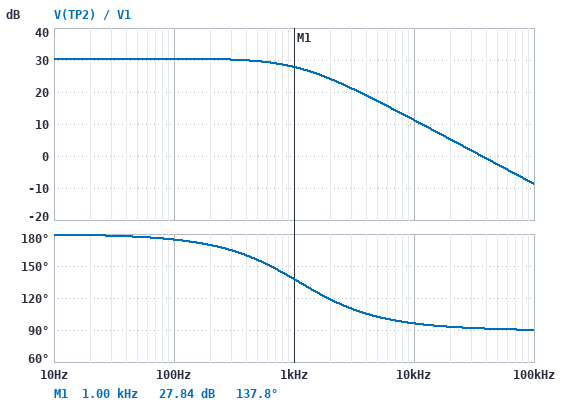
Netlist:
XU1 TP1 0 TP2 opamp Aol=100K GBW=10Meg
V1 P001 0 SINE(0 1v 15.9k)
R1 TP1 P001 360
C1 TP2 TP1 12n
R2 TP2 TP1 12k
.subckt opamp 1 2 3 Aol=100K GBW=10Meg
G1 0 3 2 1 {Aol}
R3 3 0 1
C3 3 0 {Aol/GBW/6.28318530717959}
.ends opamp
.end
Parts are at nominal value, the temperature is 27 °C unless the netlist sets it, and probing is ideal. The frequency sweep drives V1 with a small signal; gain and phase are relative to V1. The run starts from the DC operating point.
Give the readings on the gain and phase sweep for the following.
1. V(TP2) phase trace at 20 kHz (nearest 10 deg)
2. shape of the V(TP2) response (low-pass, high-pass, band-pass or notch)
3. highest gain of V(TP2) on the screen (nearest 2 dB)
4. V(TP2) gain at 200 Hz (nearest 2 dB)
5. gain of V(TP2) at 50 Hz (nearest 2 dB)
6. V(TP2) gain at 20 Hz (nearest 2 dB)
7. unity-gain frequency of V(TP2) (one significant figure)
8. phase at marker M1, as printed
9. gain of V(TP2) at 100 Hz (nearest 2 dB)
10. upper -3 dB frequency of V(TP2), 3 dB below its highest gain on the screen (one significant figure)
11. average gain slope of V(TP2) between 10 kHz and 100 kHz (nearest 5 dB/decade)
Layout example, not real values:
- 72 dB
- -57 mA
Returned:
- 90 deg
- low-pass
- 30 dB
- 30 dB
- 30 dB
- 30 dB
- 40 kHz
- 137.8 deg
- 30 dB
- 1 kHz
- -20 dB/decade
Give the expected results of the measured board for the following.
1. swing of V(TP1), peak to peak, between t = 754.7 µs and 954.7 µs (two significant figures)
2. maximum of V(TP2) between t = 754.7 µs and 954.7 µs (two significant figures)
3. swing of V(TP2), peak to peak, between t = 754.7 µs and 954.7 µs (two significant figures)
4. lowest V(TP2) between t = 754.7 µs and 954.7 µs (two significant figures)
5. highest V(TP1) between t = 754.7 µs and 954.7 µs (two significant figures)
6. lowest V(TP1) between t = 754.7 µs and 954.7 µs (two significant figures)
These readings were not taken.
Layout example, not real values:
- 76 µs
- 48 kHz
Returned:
- 7.3 mV
- 2.3 V
- 4.6 V
- -2.3 V
- 3.7 mV
- -3.7 mV
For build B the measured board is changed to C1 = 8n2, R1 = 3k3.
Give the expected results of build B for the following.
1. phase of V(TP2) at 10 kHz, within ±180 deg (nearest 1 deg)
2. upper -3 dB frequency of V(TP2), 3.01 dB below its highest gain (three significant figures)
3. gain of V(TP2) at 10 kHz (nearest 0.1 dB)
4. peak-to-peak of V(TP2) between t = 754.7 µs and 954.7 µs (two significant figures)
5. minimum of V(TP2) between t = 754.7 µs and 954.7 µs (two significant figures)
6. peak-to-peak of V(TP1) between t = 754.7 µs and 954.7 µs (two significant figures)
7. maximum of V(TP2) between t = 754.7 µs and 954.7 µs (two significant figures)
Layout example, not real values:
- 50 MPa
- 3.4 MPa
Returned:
- 99 deg
- 1.62 kHz
- -4.7 dB
- 740 mV
- -370 mV
- 1.2 mV
- 370 mV
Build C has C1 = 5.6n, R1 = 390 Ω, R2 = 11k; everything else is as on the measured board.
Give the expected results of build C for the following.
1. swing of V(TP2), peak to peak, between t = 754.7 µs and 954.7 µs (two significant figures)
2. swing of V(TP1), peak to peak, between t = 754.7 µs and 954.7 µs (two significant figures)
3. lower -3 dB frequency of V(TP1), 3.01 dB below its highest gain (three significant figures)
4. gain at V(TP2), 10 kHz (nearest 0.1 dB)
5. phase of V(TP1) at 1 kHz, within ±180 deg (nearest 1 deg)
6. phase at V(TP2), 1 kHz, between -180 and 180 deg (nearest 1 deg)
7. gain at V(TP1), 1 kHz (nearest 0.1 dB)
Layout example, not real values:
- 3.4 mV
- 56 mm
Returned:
- 9.0 V
- 14 mV
- 2.56 kHz
- 16.9 dB
- 63 deg
- 159 deg
- -51.6 dB
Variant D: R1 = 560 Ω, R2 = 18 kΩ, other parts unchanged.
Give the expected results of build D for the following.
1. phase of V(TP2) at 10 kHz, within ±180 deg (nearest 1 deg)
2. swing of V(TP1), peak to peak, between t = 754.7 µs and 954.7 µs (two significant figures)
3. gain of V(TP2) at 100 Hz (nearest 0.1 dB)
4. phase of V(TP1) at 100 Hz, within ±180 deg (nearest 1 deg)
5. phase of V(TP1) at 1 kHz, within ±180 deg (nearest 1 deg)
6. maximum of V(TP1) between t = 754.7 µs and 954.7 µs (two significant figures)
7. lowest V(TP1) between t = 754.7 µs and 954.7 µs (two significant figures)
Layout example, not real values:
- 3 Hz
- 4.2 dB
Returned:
- 94 deg
- 4.7 mV
- 30.1 dB
- 37 deg
- 31 deg
- 2.4 mV
- -2.4 mV
